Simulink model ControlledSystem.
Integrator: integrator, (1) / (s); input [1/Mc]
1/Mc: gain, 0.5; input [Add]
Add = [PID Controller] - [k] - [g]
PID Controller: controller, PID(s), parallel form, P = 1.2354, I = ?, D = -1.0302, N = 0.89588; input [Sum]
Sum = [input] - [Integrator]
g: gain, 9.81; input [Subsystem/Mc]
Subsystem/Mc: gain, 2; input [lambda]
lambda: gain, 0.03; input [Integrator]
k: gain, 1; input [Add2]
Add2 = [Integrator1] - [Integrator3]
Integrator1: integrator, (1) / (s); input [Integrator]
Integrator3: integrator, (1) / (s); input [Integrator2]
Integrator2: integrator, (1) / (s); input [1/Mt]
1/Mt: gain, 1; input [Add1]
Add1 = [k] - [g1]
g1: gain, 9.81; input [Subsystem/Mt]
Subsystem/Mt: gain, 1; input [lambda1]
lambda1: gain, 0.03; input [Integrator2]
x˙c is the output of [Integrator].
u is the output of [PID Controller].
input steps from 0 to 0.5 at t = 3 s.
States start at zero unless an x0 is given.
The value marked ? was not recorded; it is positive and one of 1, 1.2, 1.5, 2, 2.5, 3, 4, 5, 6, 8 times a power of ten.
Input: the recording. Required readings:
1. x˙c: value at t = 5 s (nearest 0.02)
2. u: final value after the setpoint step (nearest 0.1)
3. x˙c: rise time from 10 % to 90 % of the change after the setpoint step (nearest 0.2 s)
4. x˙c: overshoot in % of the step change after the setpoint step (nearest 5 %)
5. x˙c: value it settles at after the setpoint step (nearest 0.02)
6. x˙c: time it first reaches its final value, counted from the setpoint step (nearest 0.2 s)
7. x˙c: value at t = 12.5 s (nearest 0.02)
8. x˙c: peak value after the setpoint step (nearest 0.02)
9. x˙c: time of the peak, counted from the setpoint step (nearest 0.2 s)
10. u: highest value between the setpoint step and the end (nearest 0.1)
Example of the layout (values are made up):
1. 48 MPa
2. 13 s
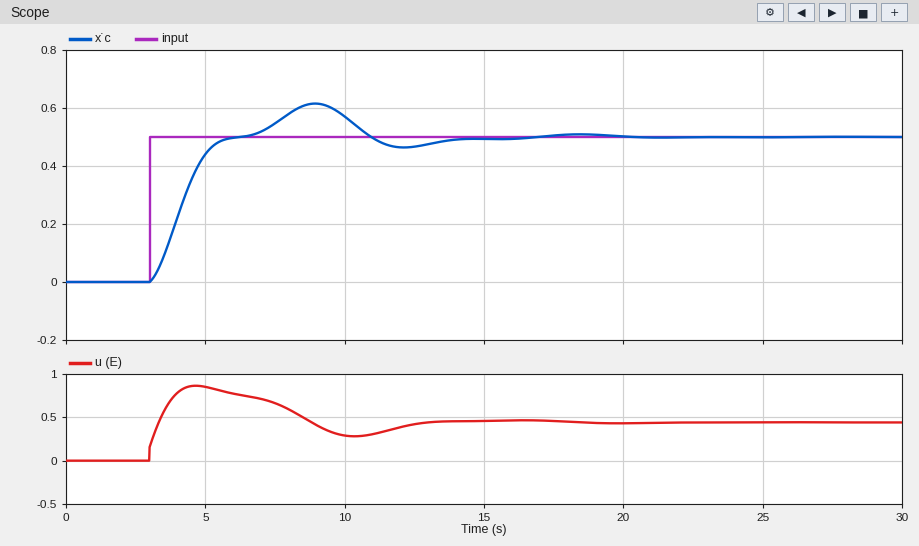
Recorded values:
1. 0.44
2. 0.4
3. 1.8 s
4. 25 %
5. 0.50
6. 3.2 s
7. 0.46
8. 0.62
9. 6.0 s
10. 0.9
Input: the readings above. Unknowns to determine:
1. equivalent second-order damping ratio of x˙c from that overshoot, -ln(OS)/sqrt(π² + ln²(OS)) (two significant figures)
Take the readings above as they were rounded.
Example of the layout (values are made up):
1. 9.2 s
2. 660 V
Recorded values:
1. 0.40
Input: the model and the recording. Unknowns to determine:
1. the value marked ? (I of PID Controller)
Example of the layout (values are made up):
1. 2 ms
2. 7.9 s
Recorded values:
1. 1.2
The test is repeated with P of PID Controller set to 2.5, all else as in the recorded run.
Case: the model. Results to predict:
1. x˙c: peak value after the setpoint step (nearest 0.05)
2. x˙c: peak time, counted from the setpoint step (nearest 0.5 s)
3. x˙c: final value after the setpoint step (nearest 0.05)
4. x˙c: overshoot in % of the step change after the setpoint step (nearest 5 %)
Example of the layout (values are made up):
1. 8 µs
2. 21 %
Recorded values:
1. 0.55
2. 5.5 s
3. 0.50
4. 15 %
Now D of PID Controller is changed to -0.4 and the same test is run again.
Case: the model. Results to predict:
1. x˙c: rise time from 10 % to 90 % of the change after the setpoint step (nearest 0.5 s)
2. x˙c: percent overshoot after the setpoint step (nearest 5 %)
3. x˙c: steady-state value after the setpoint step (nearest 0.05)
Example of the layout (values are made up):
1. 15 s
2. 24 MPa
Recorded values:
1. 2.5 s
2. 20 %
3. 0.50
